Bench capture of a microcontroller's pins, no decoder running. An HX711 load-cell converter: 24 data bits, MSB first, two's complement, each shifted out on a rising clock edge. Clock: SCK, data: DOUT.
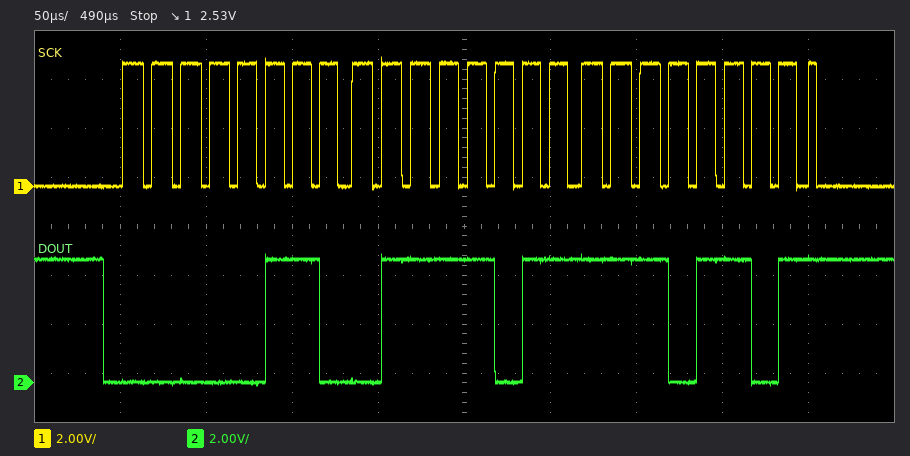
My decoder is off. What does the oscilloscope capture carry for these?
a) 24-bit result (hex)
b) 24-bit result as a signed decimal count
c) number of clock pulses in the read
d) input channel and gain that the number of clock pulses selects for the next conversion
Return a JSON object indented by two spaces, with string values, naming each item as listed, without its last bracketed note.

{
  "24-bit result": "0x067BED",
  "24-bit result as a signed decimal count": "424941",
  "number of clock pulses in the read": "25",
  "input channel and gain that the number of clock pulses selects for the next conversion": "channel A, gain 128"
}
